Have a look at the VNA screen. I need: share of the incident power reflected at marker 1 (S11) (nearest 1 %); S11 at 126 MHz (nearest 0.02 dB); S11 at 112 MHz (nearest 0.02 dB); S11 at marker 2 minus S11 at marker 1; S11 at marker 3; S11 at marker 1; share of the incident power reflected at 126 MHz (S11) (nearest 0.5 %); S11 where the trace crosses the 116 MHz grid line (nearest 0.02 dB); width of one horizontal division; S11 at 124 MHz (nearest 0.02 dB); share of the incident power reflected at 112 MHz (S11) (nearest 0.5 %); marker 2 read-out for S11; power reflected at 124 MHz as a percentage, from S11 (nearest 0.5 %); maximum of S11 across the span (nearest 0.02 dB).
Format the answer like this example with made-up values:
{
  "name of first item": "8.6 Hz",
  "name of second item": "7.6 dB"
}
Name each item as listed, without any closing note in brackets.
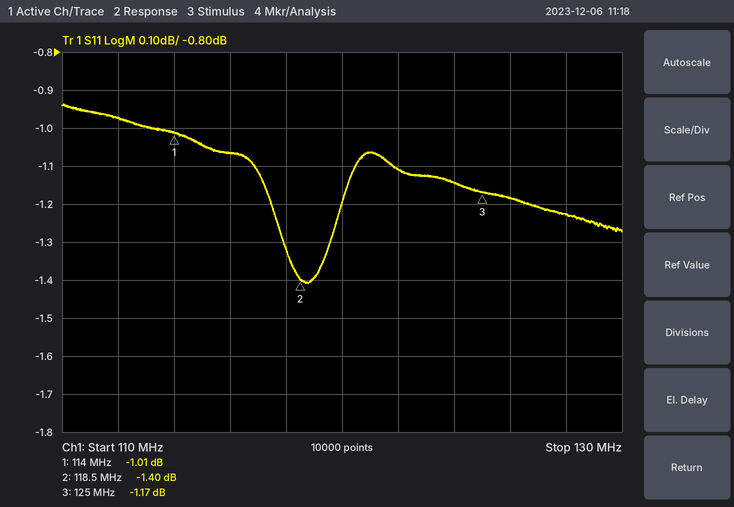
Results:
{
  "share of the incident power reflected at marker 1 (S11)": "79 %",
  "S11 at 126 MHz": "-1.18 dB",
  "S11 at 112 MHz": "-0.98 dB",
  "S11 at marker 2 minus S11 at marker 1": "-0.39 dB",
  "S11 at marker 3": "-1.17 dB",
  "S11 at marker 1": "-1.01 dB",
  "share of the incident power reflected at 126 MHz (S11)": "76.0 %",
  "S11 where the trace crosses the 116 MHz grid line": "-1.06 dB",
  "width of one horizontal division": "2 MHz",
  "S11 at 124 MHz": "-1.14 dB",
  "share of the incident power reflected at 112 MHz (S11)": "80.0 %",
  "marker 2 read-out for S11": "-1.40 dB",
  "power reflected at 124 MHz as a percentage, from S11": "77.0 %",
  "maximum of S11 across the span": "-0.94 dB"
}
